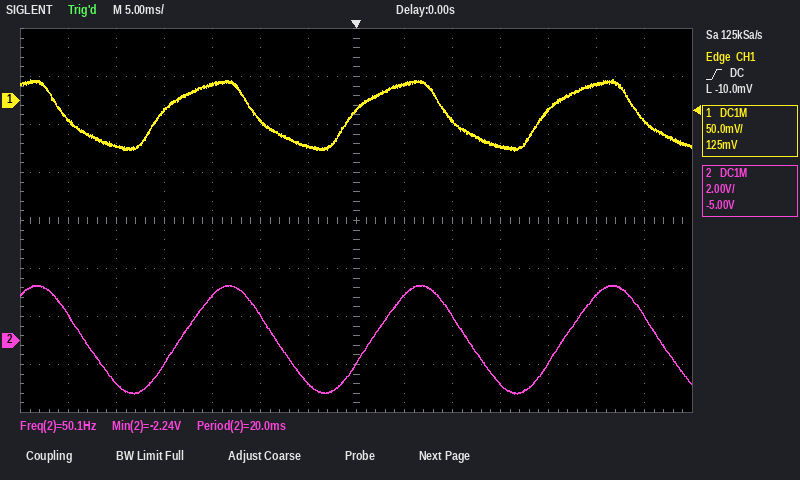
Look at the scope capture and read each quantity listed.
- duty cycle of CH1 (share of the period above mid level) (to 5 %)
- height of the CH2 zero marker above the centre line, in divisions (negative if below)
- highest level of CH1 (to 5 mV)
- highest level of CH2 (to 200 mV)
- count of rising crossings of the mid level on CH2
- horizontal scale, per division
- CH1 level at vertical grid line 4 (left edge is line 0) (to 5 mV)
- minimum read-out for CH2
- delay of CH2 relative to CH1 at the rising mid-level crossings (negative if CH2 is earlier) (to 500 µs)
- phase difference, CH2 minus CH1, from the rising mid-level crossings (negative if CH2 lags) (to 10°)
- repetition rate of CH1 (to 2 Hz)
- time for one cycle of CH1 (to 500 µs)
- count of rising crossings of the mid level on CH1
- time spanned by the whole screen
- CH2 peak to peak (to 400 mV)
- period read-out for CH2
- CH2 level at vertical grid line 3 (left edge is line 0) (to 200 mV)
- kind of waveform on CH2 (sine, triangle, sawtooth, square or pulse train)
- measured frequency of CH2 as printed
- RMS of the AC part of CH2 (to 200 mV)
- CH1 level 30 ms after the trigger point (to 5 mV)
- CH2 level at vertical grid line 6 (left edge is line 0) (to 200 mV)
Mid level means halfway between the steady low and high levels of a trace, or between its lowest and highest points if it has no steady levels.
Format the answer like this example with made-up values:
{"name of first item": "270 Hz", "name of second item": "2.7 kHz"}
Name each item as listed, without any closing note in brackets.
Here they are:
{"duty cycle of CH1 (share of the period above mid level)": "50 %", "height of the CH2 zero marker above the centre line, in divisions": "-2.5 div", "highest level of CH1": "20 mV", "highest level of CH2": "2.2 V", "count of rising crossings of the mid level on CH2": "3", "horizontal scale, per division": "5 ms", "CH1 level at vertical grid line 4 (left edge is line 0)": "15 mV", "minimum read-out for CH2": "-2.24 V", "delay of CH2 relative to CH1 at the rising mid-level crossings (negative if CH2 is earlier)": "+2.0 ms", "phase difference, CH2 minus CH1, from the rising mid-level crossings (negative if CH2 lags)": "-40°", "repetition rate of CH1": "50 Hz", "time for one cycle of CH1": "20.0 ms", "count of rising crossings of the mid level on CH1": "3", "time spanned by the whole screen": "70 ms", "CH2 peak to peak": "4.4 V", "period read-out for CH2": "20.0 ms", "CH2 level at vertical grid line 3 (left edge is line 0)": "-1.0 V", "kind of waveform on CH2": "sine", "measured frequency of CH2 as printed": "50.1 Hz", "RMS of the AC part of CH2": "1.6 V", "CH1 level 30 ms after the trigger point": "-20 mV", "CH2 level at vertical grid line 6 (left edge is line 0)": "-1.8 V"}
